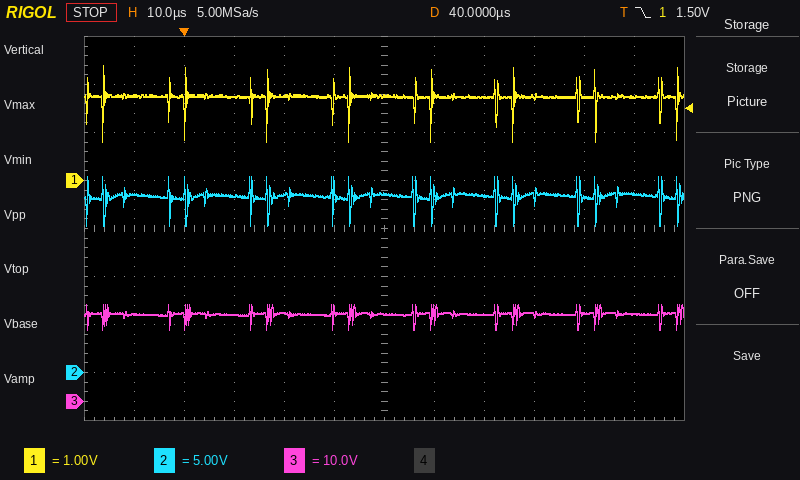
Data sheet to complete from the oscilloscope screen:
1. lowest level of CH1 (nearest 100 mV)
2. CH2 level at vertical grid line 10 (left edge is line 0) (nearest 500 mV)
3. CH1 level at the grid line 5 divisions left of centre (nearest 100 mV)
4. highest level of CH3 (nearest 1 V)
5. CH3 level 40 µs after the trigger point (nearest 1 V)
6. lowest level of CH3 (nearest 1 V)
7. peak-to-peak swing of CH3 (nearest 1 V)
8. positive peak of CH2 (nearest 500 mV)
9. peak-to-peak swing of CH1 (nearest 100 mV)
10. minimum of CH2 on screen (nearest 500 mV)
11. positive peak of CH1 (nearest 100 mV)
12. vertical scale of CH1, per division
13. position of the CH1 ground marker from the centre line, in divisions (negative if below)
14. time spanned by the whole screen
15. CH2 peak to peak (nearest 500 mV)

800 mV
18.0 V
1.8 V
20 V
18 V
15 V
5 V
20.5 V
1.6 V
15.5 V
2.4 V
1 V
+1.0 div
120 µs
5.0 V
